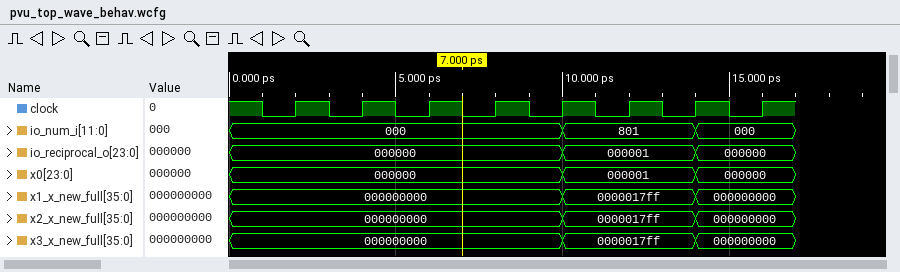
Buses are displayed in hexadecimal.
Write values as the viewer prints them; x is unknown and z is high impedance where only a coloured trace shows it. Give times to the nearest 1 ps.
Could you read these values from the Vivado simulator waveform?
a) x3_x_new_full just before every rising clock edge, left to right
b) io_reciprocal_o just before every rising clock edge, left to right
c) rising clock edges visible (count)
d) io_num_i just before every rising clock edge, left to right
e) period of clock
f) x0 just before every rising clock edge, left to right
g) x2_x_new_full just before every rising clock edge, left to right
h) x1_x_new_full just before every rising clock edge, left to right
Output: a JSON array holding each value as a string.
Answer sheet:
["000000000, 000000000, 000000000, 000000000, 000000000, 0000017ff, 0000017ff, 000000000", "000000, 000000, 000000, 000000, 000000, 000001, 000001, 000000", "8", "000, 000, 000, 000, 000, 801, 801, 000", "2 ps", "000000, 000000, 000000, 000000, 000000, 000001, 000001, 000000", "000000000, 000000000, 000000000, 000000000, 000000000, 0000017ff, 0000017ff, 000000000", "000000000, 000000000, 000000000, 000000000, 000000000, 0000017ff, 0000017ff, 000000000"]
